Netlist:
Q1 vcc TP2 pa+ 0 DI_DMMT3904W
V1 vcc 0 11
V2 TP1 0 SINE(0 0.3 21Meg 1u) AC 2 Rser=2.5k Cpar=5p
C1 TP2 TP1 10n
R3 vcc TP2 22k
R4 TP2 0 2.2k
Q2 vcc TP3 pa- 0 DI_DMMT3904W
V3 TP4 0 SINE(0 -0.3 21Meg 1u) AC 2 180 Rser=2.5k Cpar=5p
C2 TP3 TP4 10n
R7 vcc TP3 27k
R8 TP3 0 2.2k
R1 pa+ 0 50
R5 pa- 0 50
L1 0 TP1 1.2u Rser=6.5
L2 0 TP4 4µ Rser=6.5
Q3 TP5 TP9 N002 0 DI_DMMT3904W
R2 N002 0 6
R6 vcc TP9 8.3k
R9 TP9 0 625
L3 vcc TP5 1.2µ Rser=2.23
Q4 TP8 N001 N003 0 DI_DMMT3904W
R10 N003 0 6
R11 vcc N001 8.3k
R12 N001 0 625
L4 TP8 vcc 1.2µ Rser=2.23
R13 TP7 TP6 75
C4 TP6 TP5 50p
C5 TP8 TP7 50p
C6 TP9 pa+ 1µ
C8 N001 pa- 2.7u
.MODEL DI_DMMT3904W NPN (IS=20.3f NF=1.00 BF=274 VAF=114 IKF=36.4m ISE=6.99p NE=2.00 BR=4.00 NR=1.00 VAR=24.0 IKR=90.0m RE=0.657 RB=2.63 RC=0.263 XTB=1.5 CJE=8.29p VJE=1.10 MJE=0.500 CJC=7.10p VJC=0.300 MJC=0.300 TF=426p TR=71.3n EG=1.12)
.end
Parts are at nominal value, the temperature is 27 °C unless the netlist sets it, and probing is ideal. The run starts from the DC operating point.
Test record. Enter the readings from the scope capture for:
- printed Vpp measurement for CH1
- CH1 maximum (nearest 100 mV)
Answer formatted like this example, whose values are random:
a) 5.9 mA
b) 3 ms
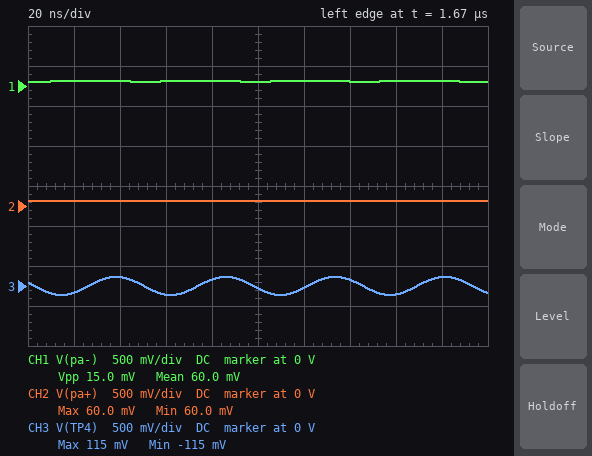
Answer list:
a) 15.0 mV
b) 100 mV
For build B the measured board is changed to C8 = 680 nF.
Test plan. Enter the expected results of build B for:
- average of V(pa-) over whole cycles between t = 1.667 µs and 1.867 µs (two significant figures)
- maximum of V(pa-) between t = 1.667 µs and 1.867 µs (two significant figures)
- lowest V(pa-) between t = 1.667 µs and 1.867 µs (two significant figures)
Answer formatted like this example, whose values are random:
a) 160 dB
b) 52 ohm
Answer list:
a) 59 mV
b) 66 mV
c) 53 mV
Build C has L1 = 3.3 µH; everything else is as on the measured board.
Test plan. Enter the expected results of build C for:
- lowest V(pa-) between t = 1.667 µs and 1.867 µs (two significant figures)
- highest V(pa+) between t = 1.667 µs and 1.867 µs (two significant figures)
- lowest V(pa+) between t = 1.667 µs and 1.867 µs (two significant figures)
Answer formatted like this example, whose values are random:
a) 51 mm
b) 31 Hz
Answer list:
a) 54 mV
b) 67 mV
c) 53 mV
